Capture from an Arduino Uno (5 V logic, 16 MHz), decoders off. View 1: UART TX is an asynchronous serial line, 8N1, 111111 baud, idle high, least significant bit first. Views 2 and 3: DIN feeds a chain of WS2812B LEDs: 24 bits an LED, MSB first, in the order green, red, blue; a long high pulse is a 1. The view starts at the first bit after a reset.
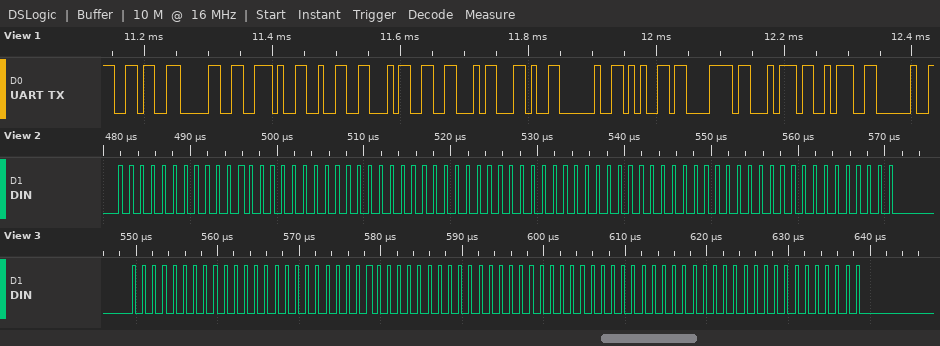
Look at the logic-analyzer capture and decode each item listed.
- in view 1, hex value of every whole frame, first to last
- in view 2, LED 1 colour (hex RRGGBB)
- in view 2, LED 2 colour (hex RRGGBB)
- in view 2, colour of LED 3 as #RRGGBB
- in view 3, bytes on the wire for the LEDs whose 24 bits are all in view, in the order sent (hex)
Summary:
0x36 0x30 0x2E 0x32 0x34 0x46 0x2C 0x20 0x65 0x78 0x74 0x3A 0x20
#100000
#000000
#000000
00 00 01 00 00 00 00 00 00
